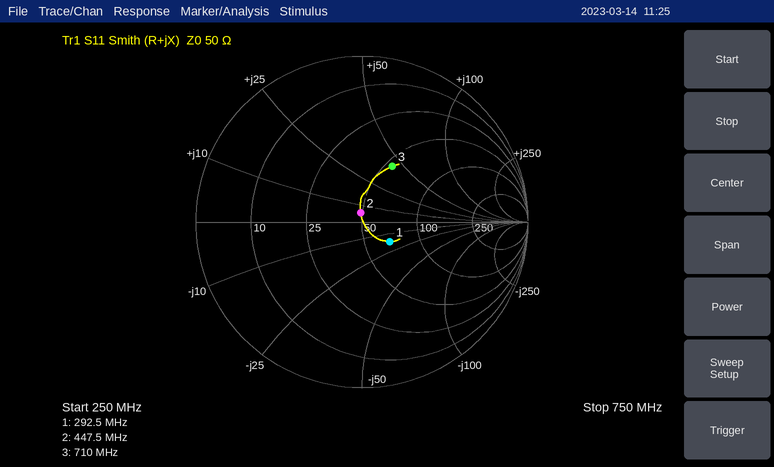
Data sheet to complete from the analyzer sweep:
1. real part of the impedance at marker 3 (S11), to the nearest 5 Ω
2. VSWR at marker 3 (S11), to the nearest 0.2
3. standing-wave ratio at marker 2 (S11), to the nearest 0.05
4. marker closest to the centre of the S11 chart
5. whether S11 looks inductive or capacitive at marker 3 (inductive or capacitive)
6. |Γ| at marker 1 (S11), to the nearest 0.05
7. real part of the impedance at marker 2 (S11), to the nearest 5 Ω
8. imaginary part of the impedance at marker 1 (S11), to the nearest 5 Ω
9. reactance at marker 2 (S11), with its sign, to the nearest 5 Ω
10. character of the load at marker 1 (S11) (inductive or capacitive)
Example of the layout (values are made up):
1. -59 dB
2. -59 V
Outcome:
1. 55 Ω
2. 2.2
3. 1.10
4. marker 2
5. inductive
6. 0.20
7. 50 Ω
8. -15 Ω
9. +5 Ω
10. capacitive
